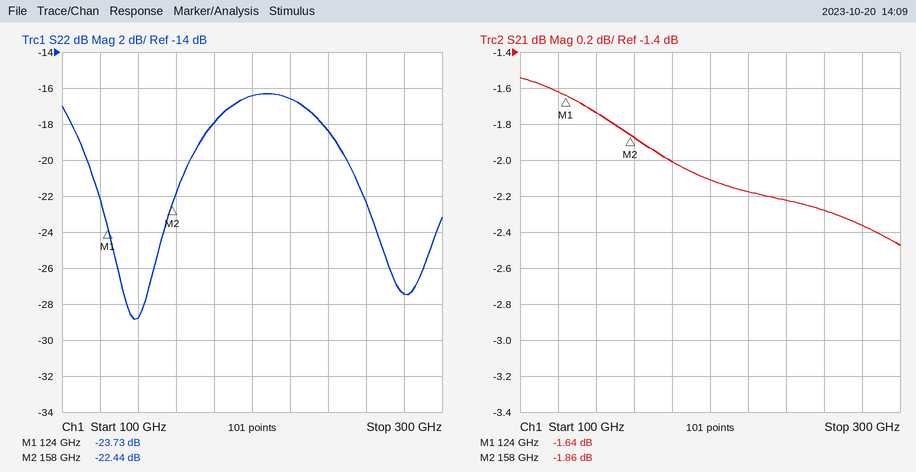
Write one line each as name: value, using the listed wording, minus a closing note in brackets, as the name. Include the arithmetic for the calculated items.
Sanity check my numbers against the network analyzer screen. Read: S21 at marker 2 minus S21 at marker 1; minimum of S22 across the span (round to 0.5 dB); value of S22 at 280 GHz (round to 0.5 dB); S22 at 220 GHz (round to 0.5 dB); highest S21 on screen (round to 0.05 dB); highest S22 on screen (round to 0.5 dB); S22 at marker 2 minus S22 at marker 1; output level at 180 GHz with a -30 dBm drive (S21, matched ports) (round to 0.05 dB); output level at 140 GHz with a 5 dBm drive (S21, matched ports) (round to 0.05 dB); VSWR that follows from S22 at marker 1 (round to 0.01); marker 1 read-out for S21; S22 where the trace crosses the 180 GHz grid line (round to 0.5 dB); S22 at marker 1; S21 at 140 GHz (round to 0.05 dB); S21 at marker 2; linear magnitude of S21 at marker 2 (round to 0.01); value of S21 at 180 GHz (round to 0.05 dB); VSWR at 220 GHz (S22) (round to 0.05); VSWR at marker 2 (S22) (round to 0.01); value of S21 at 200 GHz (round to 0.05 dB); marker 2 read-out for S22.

S21 at marker 2 minus S21 at marker 1: -1.86 − (-1.64) = -0.22 dB
minimum of S22 across the span: -29.0 dB
value of S22 at 280 GHz: -27.5 dB
S22 at 220 GHz: -16.5 dB
highest S21 on screen: -1.55 dB
highest S22 on screen: -16.5 dB
S22 at marker 2 minus S22 at marker 1: -22.44 − (-23.73) = 1.29 dB
output level at 180 GHz with a -30 dBm drive (S21, matched ports): -30 dBm + (-2.00 dB) = -32.00 dBm
output level at 140 GHz with a 5 dBm drive (S21, matched ports): 5 dBm + (-1.75 dB) = 3.25 dBm
VSWR that follows from S22 at marker 1: (1 + 0.0651)/(1 − 0.0651) ≈ 1.14
marker 1 read-out for S21: -1.64 dB
S22 where the trace crosses the 180 GHz grid line: -18.0 dB
S22 at marker 1: -23.73 dB
S21 at 140 GHz: -1.75 dB
S21 at marker 2: -1.86 dB
linear magnitude of S21 at marker 2: 10^(-1.86/20) ≈ 0.81
value of S21 at 180 GHz: -2.00 dB
VSWR at 220 GHz (S22): |Γ| = 10^(-16.5/20) = 0.1496; VSWR = (1 + 0.1496)/(1 − 0.1496) ≈ 1.35
VSWR at marker 2 (S22): (1 + 0.0755)/(1 − 0.0755) ≈ 1.16
value of S21 at 200 GHz: -2.10 dB
marker 2 read-out for S22: -22.44 dB
